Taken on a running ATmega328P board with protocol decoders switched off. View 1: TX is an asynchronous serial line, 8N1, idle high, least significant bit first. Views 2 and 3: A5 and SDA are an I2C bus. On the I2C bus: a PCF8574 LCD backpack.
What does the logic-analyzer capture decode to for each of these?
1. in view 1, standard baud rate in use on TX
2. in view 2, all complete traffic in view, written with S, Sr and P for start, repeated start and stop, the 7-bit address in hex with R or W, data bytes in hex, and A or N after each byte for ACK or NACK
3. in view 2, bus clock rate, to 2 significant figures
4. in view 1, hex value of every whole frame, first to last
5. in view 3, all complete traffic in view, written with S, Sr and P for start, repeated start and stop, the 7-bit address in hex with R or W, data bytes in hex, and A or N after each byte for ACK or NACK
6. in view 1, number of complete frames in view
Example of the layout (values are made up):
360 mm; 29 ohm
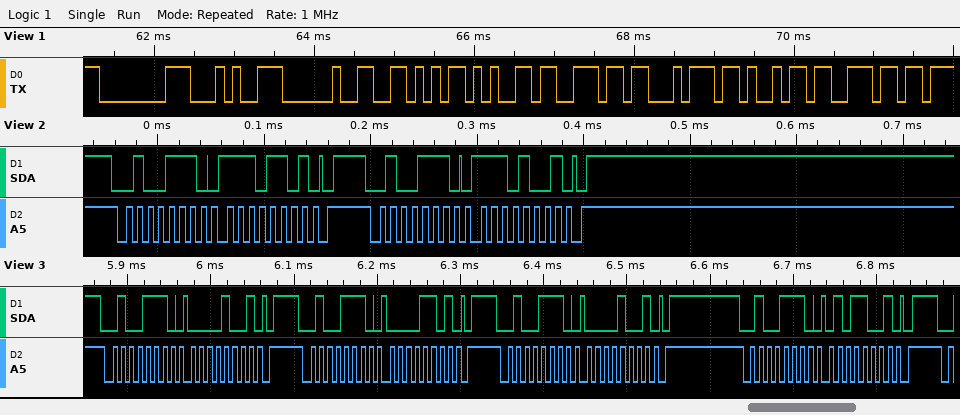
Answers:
9600 baud; S 27W A ED A P S 27W A E9 A P; 100 kHz; 80 94 20 56 65 6E 74 69 6E; S 27W A 09 A P S 27W A 0D A P S 27W A 09 A P S 27W A 59 A P; 9
